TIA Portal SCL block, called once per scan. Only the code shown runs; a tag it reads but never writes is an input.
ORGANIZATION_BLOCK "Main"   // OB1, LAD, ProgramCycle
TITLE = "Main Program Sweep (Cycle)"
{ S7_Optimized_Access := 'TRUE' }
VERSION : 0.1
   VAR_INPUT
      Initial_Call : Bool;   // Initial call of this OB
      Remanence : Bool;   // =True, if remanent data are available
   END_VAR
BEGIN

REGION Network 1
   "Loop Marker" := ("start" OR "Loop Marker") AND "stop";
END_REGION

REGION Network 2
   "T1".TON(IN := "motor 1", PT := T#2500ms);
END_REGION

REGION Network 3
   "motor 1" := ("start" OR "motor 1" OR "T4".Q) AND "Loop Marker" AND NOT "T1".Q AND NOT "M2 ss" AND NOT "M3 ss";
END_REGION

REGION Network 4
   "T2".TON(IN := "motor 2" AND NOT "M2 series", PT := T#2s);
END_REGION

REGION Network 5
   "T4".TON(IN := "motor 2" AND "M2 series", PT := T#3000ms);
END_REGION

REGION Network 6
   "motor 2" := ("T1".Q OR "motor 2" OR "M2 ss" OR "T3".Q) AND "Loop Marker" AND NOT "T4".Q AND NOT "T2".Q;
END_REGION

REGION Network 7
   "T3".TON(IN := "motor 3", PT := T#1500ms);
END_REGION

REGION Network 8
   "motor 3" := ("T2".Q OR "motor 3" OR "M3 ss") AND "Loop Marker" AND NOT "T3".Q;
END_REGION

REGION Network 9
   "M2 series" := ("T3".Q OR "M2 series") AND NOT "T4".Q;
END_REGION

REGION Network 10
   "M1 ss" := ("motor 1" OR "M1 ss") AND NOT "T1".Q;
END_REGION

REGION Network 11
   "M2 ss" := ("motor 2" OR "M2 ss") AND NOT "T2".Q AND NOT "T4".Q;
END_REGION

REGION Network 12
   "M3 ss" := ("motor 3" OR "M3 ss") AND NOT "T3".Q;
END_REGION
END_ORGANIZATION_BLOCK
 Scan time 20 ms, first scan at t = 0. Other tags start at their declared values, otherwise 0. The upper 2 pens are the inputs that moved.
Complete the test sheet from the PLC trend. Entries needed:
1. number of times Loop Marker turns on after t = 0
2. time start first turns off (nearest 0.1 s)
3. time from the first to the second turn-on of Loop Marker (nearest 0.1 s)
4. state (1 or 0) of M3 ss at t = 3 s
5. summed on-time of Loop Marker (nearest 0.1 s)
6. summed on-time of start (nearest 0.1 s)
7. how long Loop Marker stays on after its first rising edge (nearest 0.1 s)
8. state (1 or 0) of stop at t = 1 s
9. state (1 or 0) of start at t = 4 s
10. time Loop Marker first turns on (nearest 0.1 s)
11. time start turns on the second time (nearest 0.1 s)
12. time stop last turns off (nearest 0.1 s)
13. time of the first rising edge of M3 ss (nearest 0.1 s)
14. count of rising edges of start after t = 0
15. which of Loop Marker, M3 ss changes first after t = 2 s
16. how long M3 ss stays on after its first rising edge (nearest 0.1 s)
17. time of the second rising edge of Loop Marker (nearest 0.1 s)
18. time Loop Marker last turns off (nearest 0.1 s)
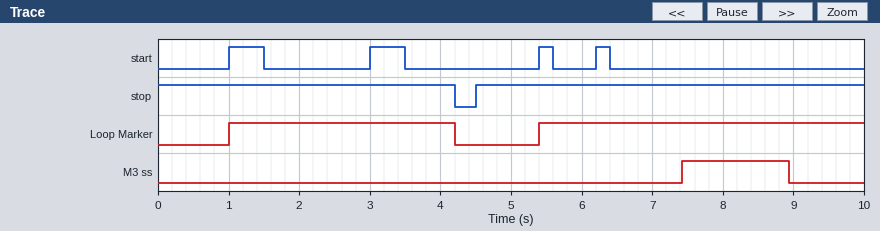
2
1.5 s
4.4 s
0
7.8 s
1.4 s
3.2 s
1
0
1.0 s
3.0 s
4.2 s
7.4 s
4
Loop Marker
1.5 s
5.4 s
4.2 s
